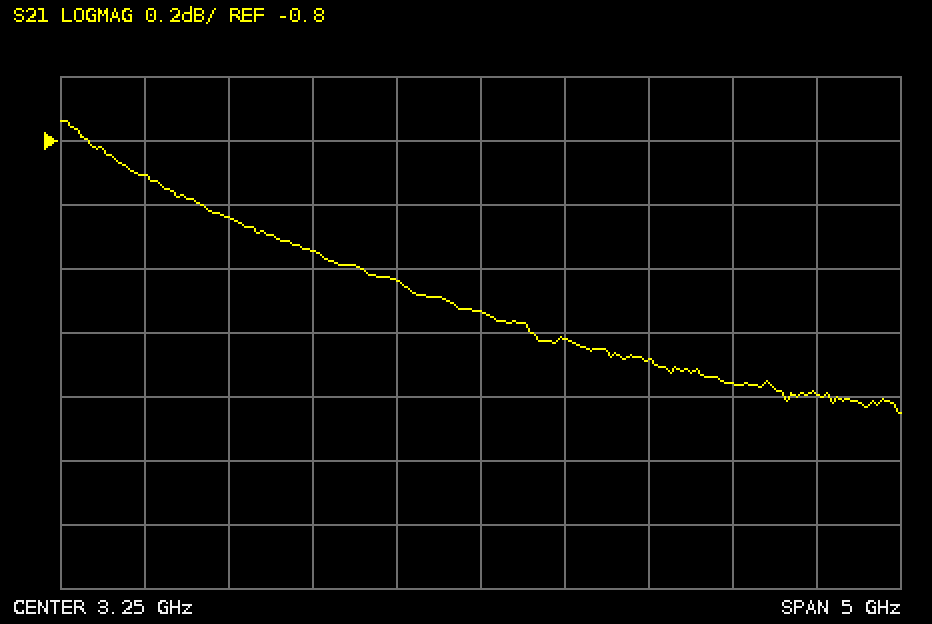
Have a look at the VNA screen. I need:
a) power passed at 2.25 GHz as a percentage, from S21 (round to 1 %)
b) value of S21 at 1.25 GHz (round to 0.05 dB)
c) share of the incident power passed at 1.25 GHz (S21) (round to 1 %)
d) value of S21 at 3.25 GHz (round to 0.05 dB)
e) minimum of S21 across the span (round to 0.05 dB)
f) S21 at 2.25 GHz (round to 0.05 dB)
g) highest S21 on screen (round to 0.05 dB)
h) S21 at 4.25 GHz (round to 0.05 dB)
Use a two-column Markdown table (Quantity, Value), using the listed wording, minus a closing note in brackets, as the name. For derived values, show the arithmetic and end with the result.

| Quantity | Value |
|---|---|
| power passed at 2.25 GHz as a percentage, from S21 | 10^(-1.15/10) ≈ 77 % |
| value of S21 at 1.25 GHz | -0.90 dB |
| share of the incident power passed at 1.25 GHz (S21) | 10^(-0.9/10) ≈ 81 % |
| value of S21 at 3.25 GHz | -1.35 dB |
| minimum of S21 across the span | -1.65 dB |
| S21 at 2.25 GHz | -1.15 dB |
| highest S21 on screen | -0.75 dB |
| S21 at 4.25 GHz | -1.50 dB |
